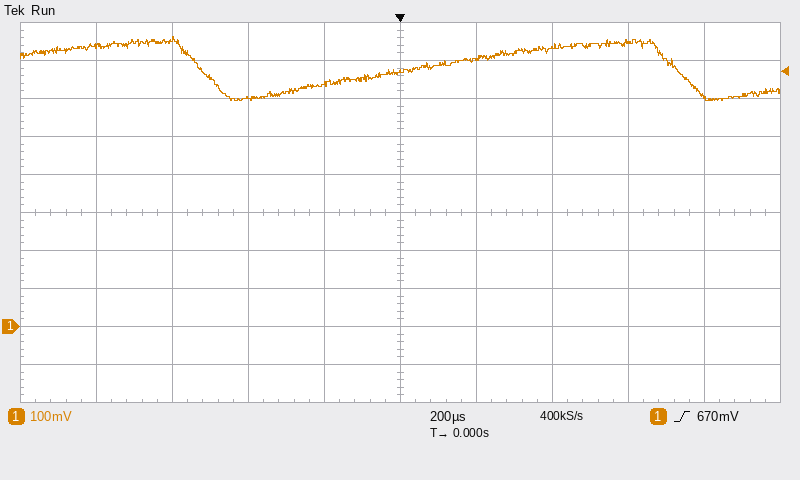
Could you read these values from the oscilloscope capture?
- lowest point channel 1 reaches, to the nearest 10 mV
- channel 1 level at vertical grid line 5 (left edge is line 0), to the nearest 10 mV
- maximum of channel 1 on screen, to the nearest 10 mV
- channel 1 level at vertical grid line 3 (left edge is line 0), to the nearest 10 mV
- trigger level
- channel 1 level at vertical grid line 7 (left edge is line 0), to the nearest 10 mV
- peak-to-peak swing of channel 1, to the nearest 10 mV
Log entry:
590 mV
670 mV
760 mV
600 mV
670 mV
740 mV
170 mV
